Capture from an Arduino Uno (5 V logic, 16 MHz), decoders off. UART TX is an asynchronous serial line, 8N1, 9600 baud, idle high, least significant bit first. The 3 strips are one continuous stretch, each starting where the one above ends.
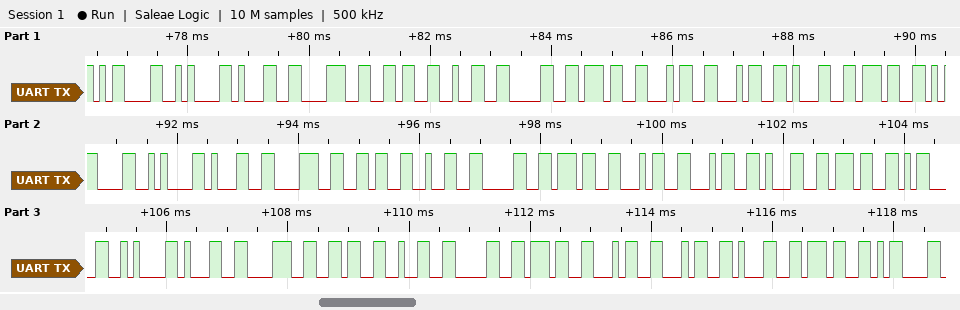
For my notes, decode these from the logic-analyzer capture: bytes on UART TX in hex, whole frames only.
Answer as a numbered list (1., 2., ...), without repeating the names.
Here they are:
1. 0x0D 0x0A 0x31 0x38 0x36 0x32 0x30 0x37 0x34 0x34 0x31 0x37 0x0D 0x0A 0x31 0x38 0x36 0x32 0x30 0x37 0x34 0x34 0x31 0x37 0x0D 0x0A 0x31 0x38 0x36 0x32 0x30 0x37 0x34 0x34 0x31 0x37 0x0D
